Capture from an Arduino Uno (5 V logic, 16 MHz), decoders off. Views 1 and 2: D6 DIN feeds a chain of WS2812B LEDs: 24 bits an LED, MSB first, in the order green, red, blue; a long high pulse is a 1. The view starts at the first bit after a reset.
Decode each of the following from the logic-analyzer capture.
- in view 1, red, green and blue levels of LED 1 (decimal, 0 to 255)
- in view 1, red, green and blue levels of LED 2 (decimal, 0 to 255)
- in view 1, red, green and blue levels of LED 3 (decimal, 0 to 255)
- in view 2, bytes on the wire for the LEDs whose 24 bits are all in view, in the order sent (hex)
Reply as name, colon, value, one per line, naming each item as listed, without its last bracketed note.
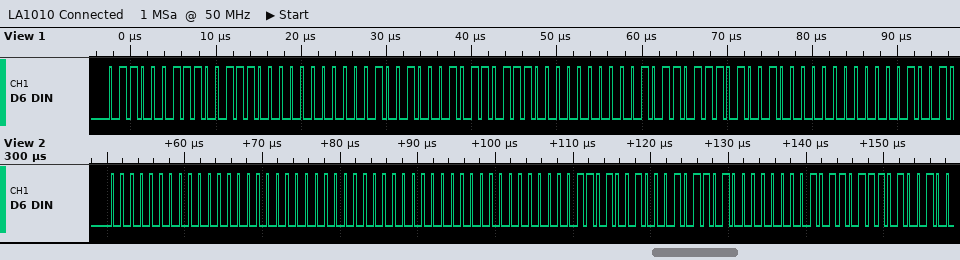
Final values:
in view 1, red, green and blue levels of LED 1: 156, 99, 0
in view 1, red, green and blue levels of LED 2: 183, 72, 0
in view 1, red, green and blue levels of LED 3: 210, 45, 0
in view 2, bytes on the wire for the LEDs whose 24 bits are all in view, in the order sent: 00 00 00 00 00 00 D2 2D 00
